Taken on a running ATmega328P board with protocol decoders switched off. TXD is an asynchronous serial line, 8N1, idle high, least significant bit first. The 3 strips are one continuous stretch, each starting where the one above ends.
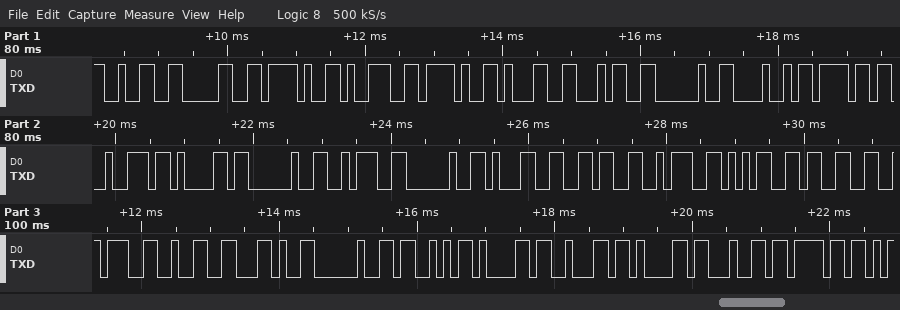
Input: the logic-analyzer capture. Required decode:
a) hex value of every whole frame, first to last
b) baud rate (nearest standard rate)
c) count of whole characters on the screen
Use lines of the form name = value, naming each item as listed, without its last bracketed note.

hex value of every whole frame, first to last = 32 30 2F 39 2F 31 34 20 48 6F 72 61 20 3A 20 31 36 3A 35 33 3A 32 2C 20 53 61 62 61 64 6F
baud rate = 9600 baud
count of whole characters on the screen = 30
